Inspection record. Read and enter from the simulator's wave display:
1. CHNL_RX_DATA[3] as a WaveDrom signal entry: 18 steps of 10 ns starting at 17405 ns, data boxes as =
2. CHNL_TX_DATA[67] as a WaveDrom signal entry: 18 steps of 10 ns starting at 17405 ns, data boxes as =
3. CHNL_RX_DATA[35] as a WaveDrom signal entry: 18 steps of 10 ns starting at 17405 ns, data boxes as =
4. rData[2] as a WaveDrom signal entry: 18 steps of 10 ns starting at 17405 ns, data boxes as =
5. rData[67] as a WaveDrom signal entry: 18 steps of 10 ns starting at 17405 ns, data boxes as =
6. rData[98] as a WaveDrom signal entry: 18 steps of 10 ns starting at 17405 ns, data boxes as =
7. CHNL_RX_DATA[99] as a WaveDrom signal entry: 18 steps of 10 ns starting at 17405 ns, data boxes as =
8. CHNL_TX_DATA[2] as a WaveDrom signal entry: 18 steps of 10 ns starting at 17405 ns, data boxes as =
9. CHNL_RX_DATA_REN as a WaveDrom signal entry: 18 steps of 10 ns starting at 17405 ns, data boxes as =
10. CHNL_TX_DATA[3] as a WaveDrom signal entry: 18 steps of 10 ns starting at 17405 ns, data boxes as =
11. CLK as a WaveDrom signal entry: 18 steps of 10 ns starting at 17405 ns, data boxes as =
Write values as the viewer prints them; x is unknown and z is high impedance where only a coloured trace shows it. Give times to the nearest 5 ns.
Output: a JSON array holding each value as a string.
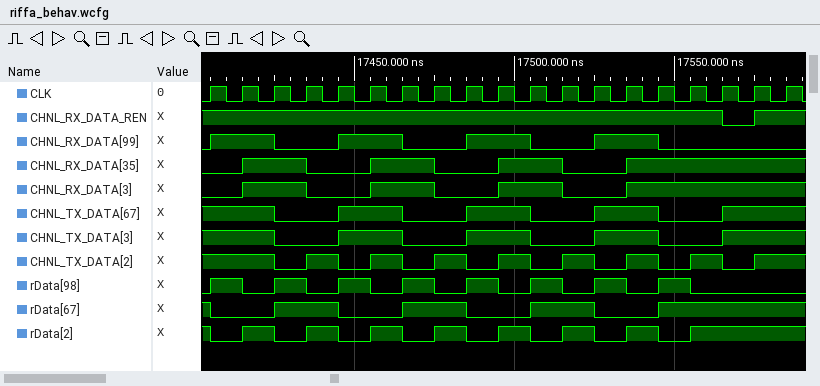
["{name: 'CHNL_RX_DATA[3]', wave: '01.0.1.0.1.0.1....'}", "{name: 'CHNL_TX_DATA[67]', wave: '1.0.1.0.1.0.1.0.1.'}", "{name: 'CHNL_RX_DATA[35]', wave: '01.0.1.0.1.0.1....'}", "{name: 'rData[2]', wave: '0101010101010101..'}", "{name: 'rData[67]', wave: '0.1.0.1.0.1.0.1...'}", "{name: 'rData[98]', wave: '1010101010101010..'}", "{name: 'CHNL_RX_DATA[99]', wave: '1.0.1.0.1.0.1.0...'}", "{name: 'CHNL_TX_DATA[2]', wave: '1.0101010101010101'}", "{name: 'CHNL_RX_DATA_REN', wave: '1...............01'}", "{name: 'CHNL_TX_DATA[3]', wave: '1.0.1.0.1.0.1.0.1.'}", "{name: 'CLK', wave: 'p.................'}"]
